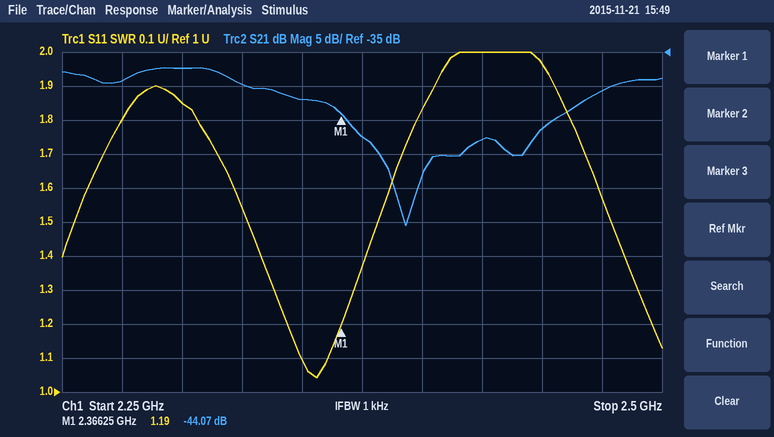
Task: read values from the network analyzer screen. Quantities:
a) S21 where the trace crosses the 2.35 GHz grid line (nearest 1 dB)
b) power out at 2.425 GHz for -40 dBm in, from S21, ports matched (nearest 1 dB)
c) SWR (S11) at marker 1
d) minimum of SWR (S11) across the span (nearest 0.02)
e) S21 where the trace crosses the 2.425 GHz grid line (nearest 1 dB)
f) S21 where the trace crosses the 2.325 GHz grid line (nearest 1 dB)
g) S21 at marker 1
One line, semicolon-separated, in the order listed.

-42 dB; -88 dBm; 1.19; 1.04; -48 dB; -40 dB; -44.07 dB
